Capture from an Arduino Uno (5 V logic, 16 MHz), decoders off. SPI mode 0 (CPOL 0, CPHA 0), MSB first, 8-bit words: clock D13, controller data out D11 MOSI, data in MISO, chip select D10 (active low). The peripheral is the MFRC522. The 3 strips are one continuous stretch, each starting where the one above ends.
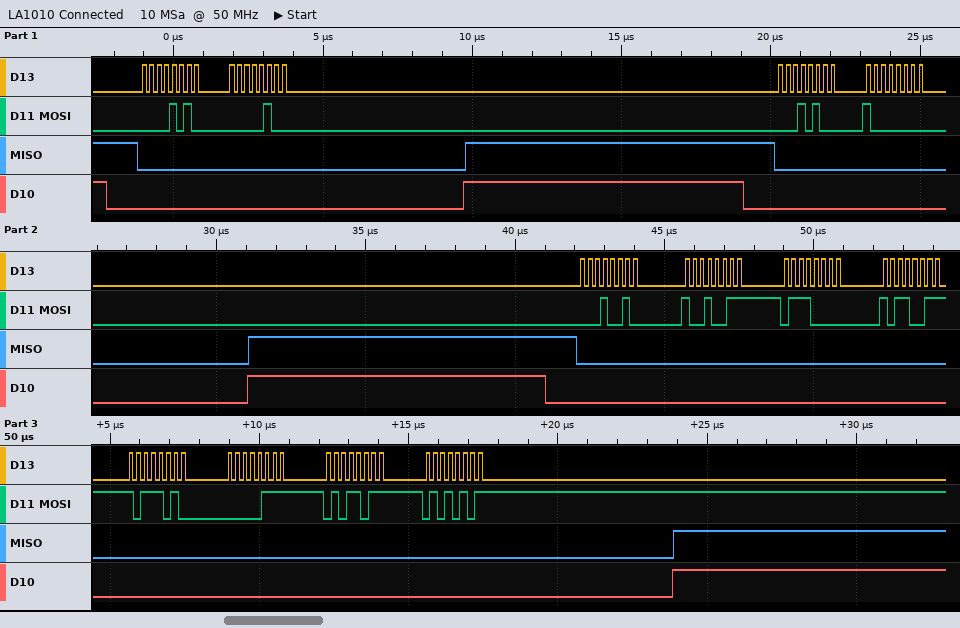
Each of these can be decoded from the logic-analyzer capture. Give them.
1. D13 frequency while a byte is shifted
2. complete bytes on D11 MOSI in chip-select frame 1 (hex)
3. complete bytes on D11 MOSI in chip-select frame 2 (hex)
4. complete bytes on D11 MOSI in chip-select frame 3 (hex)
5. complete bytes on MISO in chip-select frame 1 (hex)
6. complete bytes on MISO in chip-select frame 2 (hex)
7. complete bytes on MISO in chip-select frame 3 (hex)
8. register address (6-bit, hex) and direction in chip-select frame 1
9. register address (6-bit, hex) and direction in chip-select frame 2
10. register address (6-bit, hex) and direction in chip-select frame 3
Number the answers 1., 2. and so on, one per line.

1. 4 MHz
2. 0A 04
3. 14 80
4. 12 93 70 B3 BA 07 5B 55
5. 00 00
6. 00 00
7. 00 00 00 00 00 00 00 00
8. 0x05 write
9. 0x0A write
10. 0x09 write
